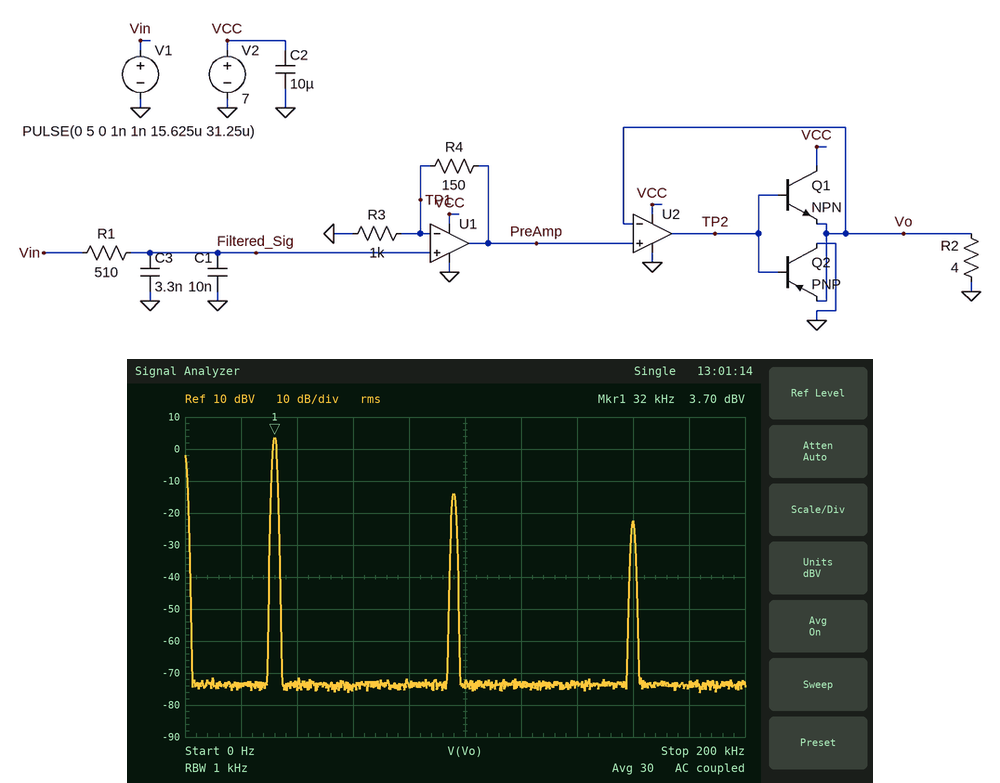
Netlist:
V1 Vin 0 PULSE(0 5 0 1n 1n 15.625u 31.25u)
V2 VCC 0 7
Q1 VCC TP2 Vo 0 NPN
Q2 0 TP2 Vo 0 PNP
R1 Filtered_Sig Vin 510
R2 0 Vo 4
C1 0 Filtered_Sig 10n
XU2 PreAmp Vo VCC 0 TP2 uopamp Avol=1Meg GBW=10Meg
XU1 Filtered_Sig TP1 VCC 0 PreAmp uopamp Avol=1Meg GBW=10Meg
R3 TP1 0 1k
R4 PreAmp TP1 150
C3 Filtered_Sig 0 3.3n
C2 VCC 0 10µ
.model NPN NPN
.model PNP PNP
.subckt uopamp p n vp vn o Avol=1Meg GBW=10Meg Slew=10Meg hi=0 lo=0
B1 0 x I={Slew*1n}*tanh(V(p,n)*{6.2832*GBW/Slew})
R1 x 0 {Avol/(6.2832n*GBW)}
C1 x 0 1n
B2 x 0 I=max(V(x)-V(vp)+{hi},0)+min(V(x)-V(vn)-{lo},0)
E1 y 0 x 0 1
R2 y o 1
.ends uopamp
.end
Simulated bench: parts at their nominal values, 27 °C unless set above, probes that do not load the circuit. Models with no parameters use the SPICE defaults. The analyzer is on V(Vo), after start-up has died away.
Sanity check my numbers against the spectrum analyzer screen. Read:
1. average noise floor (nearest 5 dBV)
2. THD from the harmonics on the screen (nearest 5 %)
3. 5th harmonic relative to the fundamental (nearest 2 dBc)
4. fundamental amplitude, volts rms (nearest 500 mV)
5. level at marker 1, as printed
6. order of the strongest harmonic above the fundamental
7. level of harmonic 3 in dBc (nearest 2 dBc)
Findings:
-75 dBV
15 %
-26 dBc
1.5 V
3.70 dBV
3
-18 dBc
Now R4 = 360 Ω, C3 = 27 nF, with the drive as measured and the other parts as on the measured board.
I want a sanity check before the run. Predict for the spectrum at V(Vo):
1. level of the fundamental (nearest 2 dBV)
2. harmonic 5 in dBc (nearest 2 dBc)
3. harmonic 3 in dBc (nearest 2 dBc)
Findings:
-2 dBV
-28 dBc
-18 dBc
